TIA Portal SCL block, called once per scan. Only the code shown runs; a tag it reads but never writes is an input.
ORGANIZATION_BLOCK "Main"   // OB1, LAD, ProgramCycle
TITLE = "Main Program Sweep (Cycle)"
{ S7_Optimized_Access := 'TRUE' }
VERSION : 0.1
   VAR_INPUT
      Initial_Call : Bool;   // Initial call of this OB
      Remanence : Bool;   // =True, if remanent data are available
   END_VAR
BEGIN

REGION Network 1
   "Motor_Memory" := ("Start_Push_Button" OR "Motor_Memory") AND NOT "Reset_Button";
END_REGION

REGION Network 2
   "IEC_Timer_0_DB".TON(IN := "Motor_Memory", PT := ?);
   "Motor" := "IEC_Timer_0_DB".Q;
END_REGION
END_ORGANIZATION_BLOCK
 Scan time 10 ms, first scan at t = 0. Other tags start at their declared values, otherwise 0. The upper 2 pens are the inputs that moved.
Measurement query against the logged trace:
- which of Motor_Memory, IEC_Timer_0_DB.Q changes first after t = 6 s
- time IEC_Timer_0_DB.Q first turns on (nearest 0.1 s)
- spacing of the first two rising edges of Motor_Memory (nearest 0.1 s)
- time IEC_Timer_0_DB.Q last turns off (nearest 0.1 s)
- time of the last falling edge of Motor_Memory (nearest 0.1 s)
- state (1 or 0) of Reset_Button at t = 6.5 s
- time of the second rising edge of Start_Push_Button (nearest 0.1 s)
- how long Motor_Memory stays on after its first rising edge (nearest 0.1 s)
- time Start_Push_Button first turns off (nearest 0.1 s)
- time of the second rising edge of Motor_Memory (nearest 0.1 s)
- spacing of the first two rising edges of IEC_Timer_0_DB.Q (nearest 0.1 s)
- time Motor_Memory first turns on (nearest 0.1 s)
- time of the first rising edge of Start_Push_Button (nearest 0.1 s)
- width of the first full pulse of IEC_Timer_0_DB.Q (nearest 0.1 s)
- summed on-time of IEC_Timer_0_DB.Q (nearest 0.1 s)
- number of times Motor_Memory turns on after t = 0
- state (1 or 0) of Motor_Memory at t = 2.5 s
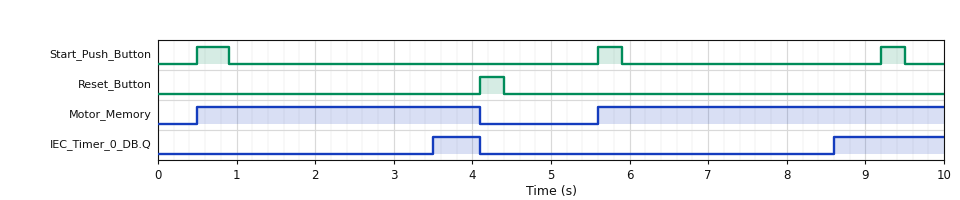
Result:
IEC_Timer_0_DB.Q
3.5 s
5.1 s
4.1 s
4.1 s
0
5.6 s
3.6 s
0.9 s
5.6 s
5.1 s
0.5 s
0.5 s
0.6 s
2.0 s
2
1
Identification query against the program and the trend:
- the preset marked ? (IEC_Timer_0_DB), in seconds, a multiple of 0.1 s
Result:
3.0 s
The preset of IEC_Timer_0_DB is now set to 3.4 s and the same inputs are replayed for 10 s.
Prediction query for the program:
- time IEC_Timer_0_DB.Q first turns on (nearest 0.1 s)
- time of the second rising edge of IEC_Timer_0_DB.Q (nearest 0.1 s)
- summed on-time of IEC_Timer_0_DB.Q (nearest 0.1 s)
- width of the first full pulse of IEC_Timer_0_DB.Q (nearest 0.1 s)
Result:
3.9 s
9.0 s
1.2 s
0.2 s
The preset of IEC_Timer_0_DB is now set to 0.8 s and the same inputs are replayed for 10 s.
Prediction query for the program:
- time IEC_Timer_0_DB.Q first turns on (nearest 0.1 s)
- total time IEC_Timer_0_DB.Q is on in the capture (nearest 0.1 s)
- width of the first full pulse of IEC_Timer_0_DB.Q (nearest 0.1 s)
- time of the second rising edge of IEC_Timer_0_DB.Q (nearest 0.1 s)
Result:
1.3 s
6.4 s
2.8 s
6.4 s
